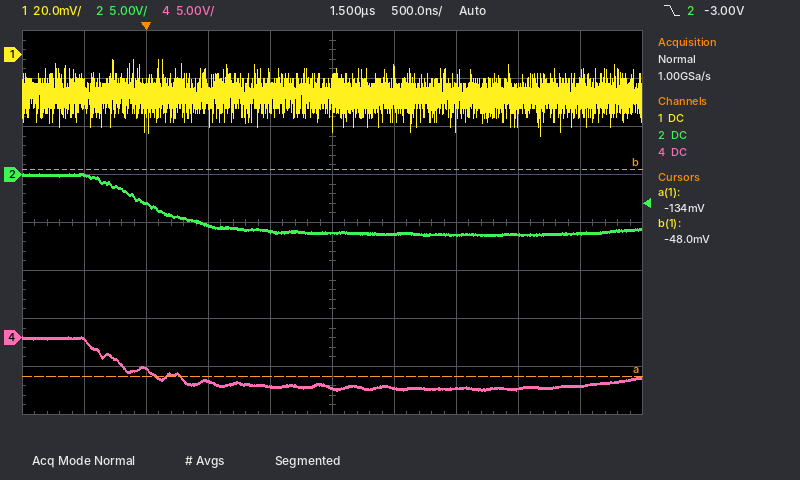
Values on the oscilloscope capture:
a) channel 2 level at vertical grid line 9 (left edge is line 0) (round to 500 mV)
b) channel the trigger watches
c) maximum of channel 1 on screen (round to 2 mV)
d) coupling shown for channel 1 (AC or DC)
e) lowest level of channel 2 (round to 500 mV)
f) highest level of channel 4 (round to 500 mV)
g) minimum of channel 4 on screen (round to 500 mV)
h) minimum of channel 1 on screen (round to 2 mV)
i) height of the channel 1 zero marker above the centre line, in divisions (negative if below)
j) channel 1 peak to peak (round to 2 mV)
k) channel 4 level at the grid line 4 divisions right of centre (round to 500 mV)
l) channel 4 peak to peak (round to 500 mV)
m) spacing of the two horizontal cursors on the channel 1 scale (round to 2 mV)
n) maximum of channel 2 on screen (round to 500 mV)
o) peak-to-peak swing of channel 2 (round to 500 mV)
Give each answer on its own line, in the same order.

-6.0 V
channel 2
-2 mV
DC
-6.5 V
0.0 V
-5.5 V
-34 mV
+3.5 div
32 mV
-5.0 V
5.5 V
86 mV
0.0 V
6.5 V
